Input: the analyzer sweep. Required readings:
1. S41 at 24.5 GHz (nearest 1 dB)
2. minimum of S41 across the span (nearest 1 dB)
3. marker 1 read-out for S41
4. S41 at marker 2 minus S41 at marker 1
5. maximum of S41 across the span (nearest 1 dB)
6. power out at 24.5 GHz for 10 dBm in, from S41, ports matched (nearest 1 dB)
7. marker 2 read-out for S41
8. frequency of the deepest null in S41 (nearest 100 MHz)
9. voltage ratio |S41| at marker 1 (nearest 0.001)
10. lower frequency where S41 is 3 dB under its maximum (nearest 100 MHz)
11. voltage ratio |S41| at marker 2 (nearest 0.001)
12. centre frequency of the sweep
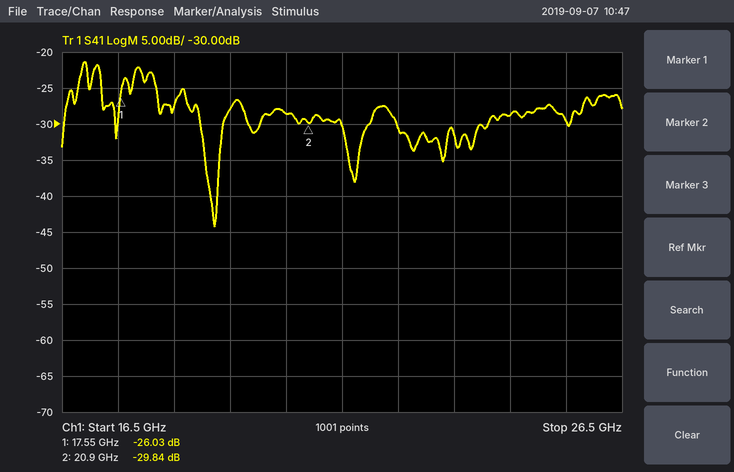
-29 dB
-44 dB
-26.03 dB
-3.81 dB
-21 dB
-19 dBm
-29.84 dB
19.2 GHz
0.050
16.8 GHz
0.032
21.5 GHz
